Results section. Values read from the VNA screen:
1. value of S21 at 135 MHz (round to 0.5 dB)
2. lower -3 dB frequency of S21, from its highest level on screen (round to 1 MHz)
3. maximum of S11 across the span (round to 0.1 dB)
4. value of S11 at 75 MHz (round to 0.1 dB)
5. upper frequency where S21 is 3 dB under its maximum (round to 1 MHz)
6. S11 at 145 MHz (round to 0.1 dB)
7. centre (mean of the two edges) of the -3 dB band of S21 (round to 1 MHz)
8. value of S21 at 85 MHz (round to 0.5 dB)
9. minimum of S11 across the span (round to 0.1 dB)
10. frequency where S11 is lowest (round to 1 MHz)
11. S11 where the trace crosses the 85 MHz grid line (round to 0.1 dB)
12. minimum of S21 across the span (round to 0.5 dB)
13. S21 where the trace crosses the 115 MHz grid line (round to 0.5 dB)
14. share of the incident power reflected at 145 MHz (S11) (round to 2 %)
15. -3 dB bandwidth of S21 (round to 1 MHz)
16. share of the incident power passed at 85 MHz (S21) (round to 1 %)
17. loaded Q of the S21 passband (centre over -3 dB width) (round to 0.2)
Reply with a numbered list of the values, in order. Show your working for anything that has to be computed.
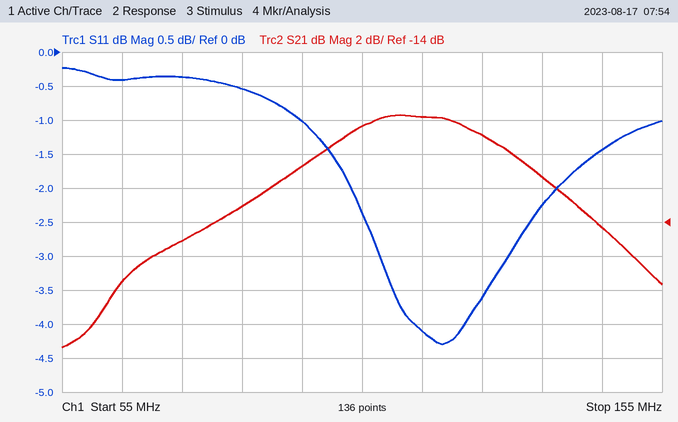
1. -11.5 dB
2. 95 MHz
3. -0.2 dB
4. -0.4 dB
5. 133 MHz
6. -1.4 dB
7. 114 MHz
8. -13.0 dB
9. -4.3 dB
10. 118 MHz
11. -0.5 dB
12. -21.5 dB
13. -8.0 dB
14. 10^(-1.4/10) ≈ 72 %
15. 133 MHz − 95 MHz = 38 MHz
16. 10^(-13/10) ≈ 5 %
17. 114 MHz / 38 MHz ≈ 3.0
